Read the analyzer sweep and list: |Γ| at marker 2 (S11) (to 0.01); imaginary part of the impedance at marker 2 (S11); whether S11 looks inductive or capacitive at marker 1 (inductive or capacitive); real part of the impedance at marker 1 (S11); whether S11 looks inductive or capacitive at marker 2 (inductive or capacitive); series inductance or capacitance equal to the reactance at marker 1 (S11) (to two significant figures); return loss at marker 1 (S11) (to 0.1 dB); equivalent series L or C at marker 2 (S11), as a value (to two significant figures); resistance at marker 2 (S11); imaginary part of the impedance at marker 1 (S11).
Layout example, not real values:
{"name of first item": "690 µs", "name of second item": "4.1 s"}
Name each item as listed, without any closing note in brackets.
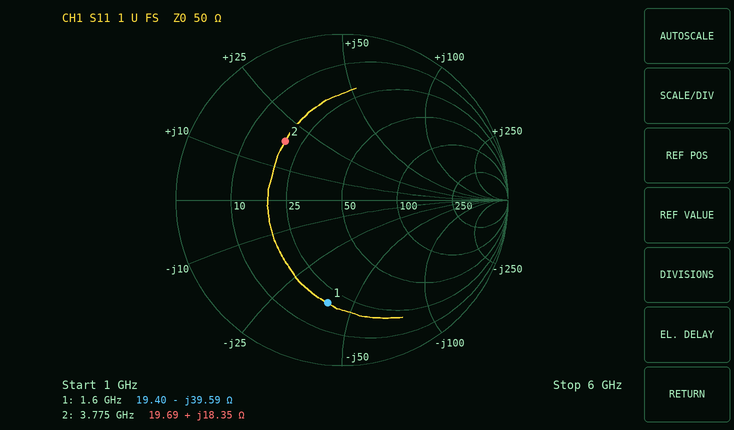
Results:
{"|Γ| at marker 2 (S11)": "0.49", "imaginary part of the impedance at marker 2": "+18.35 Ω", "whether S11 looks inductive or capacitive at marker 1": "capacitive", "real part of the impedance at marker 1": "19.40 Ω", "whether S11 looks inductive or capacitive at marker 2": "inductive", "series inductance or capacitance equal to the reactance at marker 1 (S11)": "2.5 pF", "return loss at marker 1 (S11)": "4.1 dB", "equivalent series L or C at marker 2 (S11), as a value": "770 pH", "resistance at marker 2": "19.69 Ω", "imaginary part of the impedance at marker 1": "-39.59 Ω"}
